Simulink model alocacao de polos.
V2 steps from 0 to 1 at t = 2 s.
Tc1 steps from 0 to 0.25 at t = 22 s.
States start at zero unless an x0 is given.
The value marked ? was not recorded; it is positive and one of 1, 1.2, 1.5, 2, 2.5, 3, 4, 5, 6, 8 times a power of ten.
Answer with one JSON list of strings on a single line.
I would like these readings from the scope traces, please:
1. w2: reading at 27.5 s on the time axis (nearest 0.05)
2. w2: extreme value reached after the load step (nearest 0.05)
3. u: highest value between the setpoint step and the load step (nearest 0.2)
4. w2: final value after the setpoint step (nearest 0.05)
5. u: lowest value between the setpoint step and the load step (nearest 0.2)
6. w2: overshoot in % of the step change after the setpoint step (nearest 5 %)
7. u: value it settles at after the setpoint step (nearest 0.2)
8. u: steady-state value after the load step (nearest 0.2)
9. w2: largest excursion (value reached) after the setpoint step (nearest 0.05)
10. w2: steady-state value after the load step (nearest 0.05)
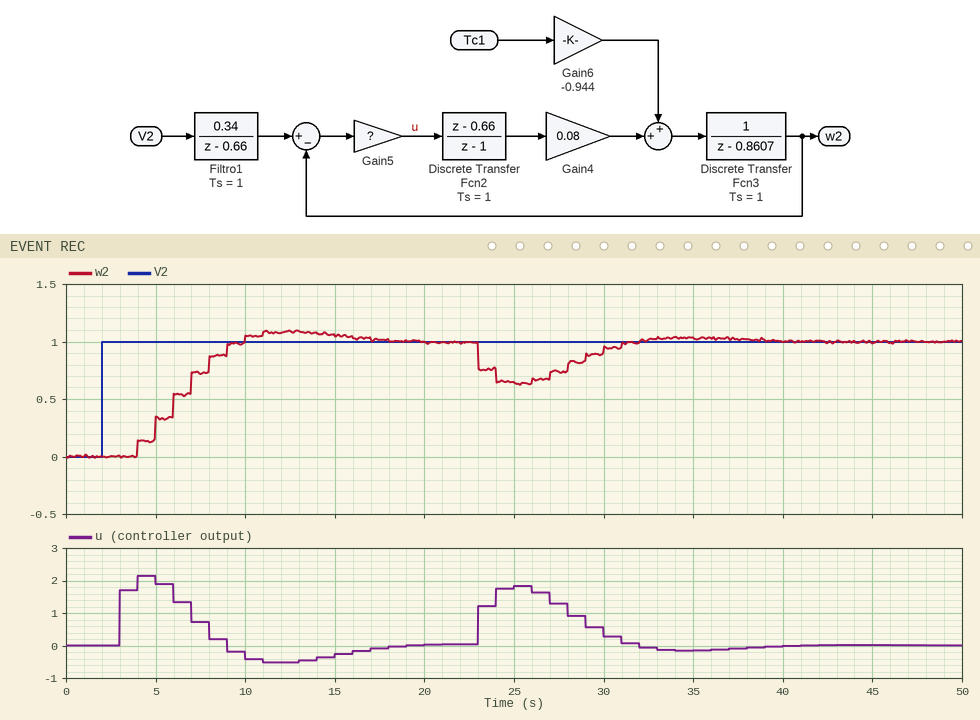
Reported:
["0.75", "0.65", "2.2", "1.00", "-0.6", "10 %", "0.0", "0.0", "1.10", "1.00"]
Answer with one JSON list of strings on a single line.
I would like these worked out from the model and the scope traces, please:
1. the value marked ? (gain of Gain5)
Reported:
["5"]
